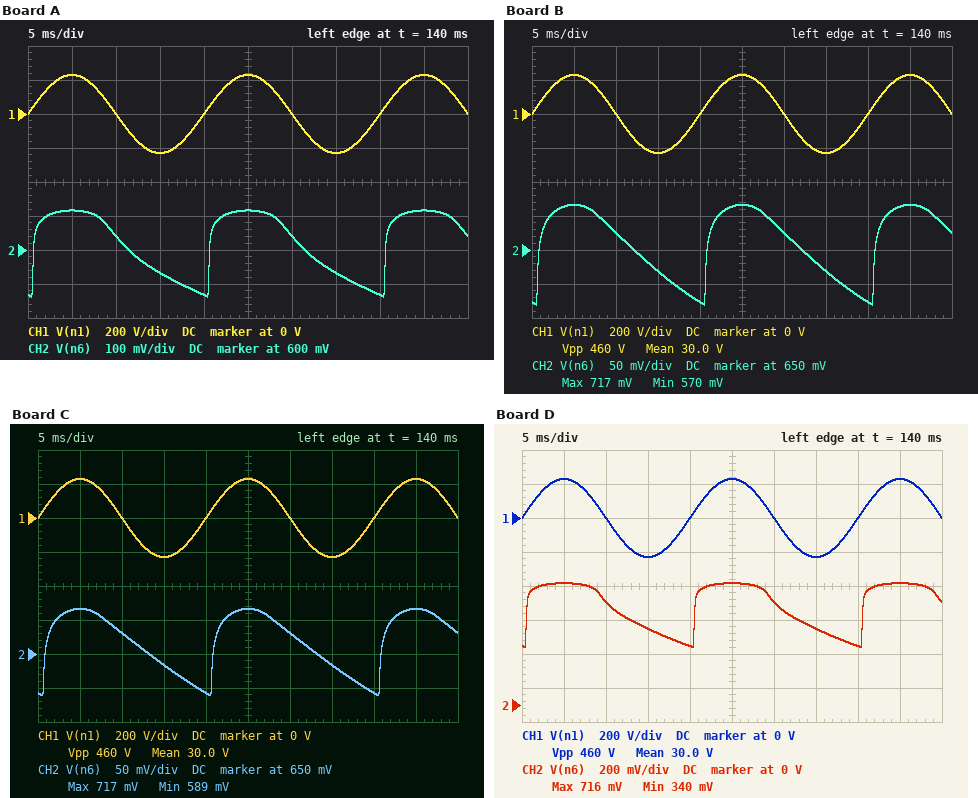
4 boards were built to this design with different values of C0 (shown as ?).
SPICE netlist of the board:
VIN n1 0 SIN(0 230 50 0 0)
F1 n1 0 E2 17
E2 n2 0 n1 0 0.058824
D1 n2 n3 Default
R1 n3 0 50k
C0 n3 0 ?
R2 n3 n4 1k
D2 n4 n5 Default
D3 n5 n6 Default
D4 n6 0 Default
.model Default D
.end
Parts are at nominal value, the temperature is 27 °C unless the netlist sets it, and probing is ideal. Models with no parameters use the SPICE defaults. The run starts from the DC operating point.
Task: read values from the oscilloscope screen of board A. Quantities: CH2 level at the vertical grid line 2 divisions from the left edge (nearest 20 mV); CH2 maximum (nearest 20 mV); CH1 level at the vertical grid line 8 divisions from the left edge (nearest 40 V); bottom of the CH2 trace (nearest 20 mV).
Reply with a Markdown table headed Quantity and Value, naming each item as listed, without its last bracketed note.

| Quantity | Value |
|---|---|
| CH2 level at the vertical grid line 2 divisions from the left edge | 640 mV |
| CH2 maximum | 720 mV |
| CH1 level at the vertical grid line 8 divisions from the left edge | 0 V |
| bottom of the CH2 trace | 460 mV |
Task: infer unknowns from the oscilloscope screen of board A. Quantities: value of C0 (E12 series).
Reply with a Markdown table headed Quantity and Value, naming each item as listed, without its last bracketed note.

| Quantity | Value |
|---|---|
| value of C0 | 820 nF |
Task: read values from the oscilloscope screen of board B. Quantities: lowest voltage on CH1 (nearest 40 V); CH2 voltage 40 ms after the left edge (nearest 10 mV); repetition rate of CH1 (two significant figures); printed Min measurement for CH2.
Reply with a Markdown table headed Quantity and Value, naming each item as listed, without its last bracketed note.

| Quantity | Value |
|---|---|
| lowest voltage on CH1 | -240 V |
| CH2 voltage 40 ms after the left edge | 570 mV |
| repetition rate of CH1 | 50 Hz |
| printed Min measurement for CH2 | 570 mV |
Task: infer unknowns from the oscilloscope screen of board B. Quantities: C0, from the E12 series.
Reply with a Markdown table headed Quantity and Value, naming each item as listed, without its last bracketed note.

| Quantity | Value |
|---|---|
| C0, from the E12 series | 2.2 µF |
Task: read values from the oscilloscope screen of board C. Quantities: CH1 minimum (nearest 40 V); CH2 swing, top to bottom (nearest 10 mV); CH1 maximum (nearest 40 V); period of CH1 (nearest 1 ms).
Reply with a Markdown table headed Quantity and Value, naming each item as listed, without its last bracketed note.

| Quantity | Value |
|---|---|
| CH1 minimum | -240 V |
| CH2 swing, top to bottom | 130 mV |
| CH1 maximum | 240 V |
| period of CH1 | 20 ms |
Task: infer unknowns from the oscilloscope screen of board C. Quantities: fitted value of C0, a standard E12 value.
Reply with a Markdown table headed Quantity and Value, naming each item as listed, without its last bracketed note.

| Quantity | Value |
|---|---|
| fitted value of C0, a standard E12 value | 2.7 µF |
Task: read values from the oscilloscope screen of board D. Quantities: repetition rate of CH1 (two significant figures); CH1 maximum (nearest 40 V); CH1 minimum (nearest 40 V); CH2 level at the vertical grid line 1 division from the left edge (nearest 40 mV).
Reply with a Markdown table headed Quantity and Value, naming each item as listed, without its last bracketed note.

| Quantity | Value |
|---|---|
| repetition rate of CH1 | 50 Hz |
| CH1 maximum | 240 V |
| CH1 minimum | -240 V |
| CH2 level at the vertical grid line 1 division from the left edge | 720 mV |
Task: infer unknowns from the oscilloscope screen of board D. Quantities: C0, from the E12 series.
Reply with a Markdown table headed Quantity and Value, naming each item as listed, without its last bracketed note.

| Quantity | Value |
|---|---|
| C0, from the E12 series | 390 nF |
